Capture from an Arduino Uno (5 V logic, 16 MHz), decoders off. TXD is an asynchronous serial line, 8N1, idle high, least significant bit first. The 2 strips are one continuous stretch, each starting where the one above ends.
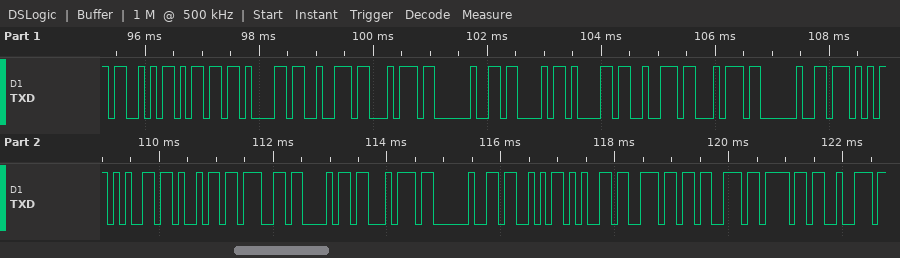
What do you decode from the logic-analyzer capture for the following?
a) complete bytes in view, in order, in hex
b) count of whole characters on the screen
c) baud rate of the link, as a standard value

53 6D 61 72 74 20 43 61 72 74 20 57 65 69 67 68 74 20 53 65 6E 73 6F 72
24
9600 baud
